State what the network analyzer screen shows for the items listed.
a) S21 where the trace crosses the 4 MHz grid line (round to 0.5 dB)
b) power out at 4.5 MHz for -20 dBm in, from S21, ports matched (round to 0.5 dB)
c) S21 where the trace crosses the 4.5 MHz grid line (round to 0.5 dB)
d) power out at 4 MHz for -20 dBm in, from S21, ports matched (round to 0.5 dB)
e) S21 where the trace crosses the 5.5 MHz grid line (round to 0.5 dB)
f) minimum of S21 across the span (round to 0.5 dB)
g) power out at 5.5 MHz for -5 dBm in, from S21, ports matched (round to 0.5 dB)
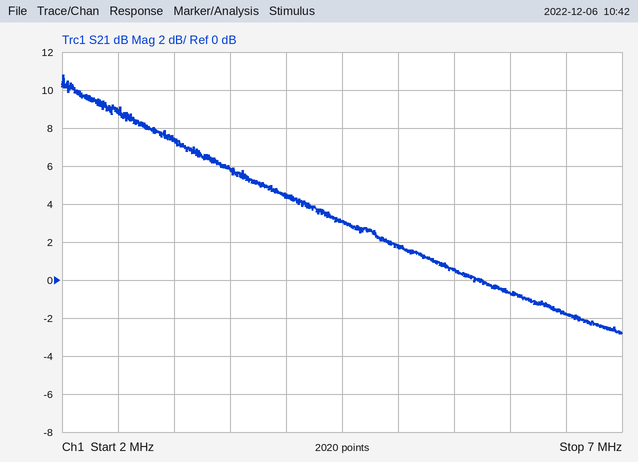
4.5 dB
-17.0 dBm
3.0 dB
-15.5 dBm
0.5 dB
-3.0 dB
-4.5 dBm
